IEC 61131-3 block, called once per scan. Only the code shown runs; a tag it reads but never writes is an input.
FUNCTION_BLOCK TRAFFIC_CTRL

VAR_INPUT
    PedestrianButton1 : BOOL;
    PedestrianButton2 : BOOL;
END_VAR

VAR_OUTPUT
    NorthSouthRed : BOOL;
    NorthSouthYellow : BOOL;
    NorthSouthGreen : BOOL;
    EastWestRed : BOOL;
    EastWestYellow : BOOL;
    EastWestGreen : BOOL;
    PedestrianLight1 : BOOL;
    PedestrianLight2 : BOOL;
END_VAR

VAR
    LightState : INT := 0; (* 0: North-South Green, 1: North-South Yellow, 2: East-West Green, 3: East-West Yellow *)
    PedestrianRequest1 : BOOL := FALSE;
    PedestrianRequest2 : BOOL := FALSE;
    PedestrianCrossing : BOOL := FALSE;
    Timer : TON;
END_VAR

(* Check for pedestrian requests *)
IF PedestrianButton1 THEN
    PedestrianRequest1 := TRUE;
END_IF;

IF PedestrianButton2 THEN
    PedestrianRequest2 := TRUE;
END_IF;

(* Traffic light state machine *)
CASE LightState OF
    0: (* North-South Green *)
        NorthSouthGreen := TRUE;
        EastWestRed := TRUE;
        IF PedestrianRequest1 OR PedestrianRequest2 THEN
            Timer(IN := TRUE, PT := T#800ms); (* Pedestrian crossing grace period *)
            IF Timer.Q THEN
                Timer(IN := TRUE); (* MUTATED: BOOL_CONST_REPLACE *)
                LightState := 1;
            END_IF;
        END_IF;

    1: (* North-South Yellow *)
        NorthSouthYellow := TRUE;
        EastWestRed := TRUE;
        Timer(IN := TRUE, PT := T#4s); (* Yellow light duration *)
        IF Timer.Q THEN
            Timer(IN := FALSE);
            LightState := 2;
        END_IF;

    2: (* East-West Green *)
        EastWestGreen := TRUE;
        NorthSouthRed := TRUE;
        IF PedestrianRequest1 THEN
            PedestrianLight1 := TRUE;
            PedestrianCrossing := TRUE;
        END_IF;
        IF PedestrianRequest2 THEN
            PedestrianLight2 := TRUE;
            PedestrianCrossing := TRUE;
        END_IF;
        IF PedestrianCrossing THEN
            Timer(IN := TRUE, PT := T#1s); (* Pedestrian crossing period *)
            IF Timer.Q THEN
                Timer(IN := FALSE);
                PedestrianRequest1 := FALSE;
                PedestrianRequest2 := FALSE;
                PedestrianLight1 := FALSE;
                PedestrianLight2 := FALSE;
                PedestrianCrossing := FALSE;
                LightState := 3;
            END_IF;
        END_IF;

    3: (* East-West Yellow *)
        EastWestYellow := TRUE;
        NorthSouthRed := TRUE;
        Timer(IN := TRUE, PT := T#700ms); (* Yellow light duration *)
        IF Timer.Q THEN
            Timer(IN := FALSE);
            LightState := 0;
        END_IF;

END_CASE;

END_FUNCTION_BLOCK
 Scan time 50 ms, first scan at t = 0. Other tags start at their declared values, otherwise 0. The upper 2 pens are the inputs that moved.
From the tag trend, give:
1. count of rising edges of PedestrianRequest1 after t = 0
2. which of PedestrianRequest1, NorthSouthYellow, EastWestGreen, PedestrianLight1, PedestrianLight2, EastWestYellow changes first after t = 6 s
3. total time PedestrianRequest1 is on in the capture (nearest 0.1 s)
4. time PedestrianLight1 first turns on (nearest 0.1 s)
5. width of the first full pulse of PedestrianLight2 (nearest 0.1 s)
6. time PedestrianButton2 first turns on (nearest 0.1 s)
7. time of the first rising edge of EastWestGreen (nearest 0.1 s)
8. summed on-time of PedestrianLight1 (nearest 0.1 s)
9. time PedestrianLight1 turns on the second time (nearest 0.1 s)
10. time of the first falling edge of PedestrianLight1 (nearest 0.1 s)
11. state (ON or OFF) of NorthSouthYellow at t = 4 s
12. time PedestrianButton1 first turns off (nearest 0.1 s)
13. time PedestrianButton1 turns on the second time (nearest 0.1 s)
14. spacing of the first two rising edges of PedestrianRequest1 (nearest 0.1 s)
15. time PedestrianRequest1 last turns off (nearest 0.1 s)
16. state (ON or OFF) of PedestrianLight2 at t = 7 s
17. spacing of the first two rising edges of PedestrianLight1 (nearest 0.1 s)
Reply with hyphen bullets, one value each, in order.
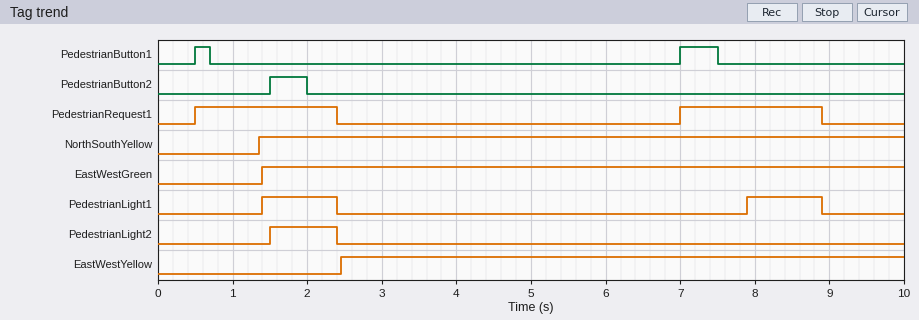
- 2
- PedestrianRequest1
- 3.8 s
- 1.4 s
- 0.9 s
- 1.5 s
- 1.4 s
- 2.0 s
- 7.9 s
- 2.4 s
- ON
- 0.7 s
- 7.0 s
- 6.5 s
- 8.9 s
- OFF
- 6.5 s
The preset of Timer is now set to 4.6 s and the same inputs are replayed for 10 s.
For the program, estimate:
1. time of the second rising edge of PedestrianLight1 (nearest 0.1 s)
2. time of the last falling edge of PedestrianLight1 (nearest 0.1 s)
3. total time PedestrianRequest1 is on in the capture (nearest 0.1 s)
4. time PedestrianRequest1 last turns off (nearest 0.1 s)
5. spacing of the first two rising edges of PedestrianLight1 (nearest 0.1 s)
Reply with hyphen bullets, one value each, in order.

- 8.0 s
- 9.0 s
- 3.9 s
- 9.0 s
- 6.6 s
